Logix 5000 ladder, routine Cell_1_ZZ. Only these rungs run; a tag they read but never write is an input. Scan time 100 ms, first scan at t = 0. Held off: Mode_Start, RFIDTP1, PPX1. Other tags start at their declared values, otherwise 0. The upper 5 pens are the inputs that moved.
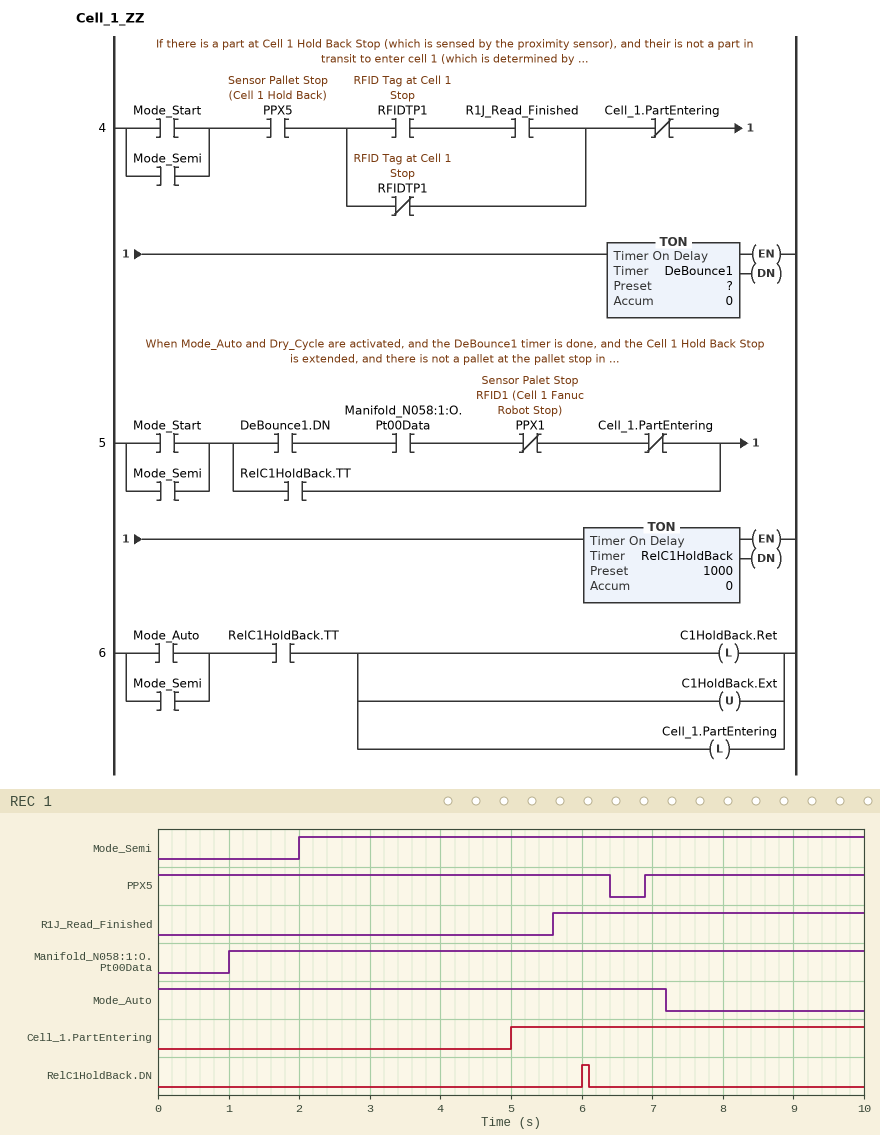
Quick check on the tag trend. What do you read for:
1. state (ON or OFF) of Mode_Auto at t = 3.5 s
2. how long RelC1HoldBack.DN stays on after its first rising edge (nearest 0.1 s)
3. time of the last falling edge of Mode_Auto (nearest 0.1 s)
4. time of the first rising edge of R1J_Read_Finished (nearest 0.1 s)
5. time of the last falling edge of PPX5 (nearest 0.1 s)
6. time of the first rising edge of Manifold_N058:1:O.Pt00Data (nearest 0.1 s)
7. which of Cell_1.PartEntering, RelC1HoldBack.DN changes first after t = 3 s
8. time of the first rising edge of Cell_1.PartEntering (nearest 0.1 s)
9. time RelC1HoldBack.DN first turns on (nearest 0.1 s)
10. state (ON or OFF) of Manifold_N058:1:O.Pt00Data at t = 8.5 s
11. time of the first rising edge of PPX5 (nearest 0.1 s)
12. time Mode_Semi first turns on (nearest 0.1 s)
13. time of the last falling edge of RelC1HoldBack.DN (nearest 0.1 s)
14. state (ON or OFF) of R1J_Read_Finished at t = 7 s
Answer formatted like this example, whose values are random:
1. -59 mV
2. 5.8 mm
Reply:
1. ON
2. 0.1 s
3. 7.2 s
4. 5.6 s
5. 6.4 s
6. 1.0 s
7. Cell_1.PartEntering
8. 5.0 s
9. 6.0 s
10. ON
11. 6.9 s
12. 2.0 s
13. 6.1 s
14. ON
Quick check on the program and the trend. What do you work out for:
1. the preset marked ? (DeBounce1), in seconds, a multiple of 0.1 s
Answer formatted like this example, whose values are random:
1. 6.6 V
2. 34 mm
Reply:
1. 3.0 s
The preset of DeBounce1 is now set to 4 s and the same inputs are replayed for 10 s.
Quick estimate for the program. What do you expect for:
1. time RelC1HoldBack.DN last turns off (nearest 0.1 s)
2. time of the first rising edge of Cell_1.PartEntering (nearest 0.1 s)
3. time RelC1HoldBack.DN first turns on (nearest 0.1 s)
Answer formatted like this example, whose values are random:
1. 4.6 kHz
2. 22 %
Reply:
1. 7.1 s
2. 6.0 s
3. 7.0 s
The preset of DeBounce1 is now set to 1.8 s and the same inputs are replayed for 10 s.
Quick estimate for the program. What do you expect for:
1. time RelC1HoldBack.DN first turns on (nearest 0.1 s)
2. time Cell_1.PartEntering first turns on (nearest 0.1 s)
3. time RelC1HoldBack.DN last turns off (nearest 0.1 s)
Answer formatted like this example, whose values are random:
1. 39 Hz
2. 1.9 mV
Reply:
1. 4.8 s
2. 3.8 s
3. 4.9 s
